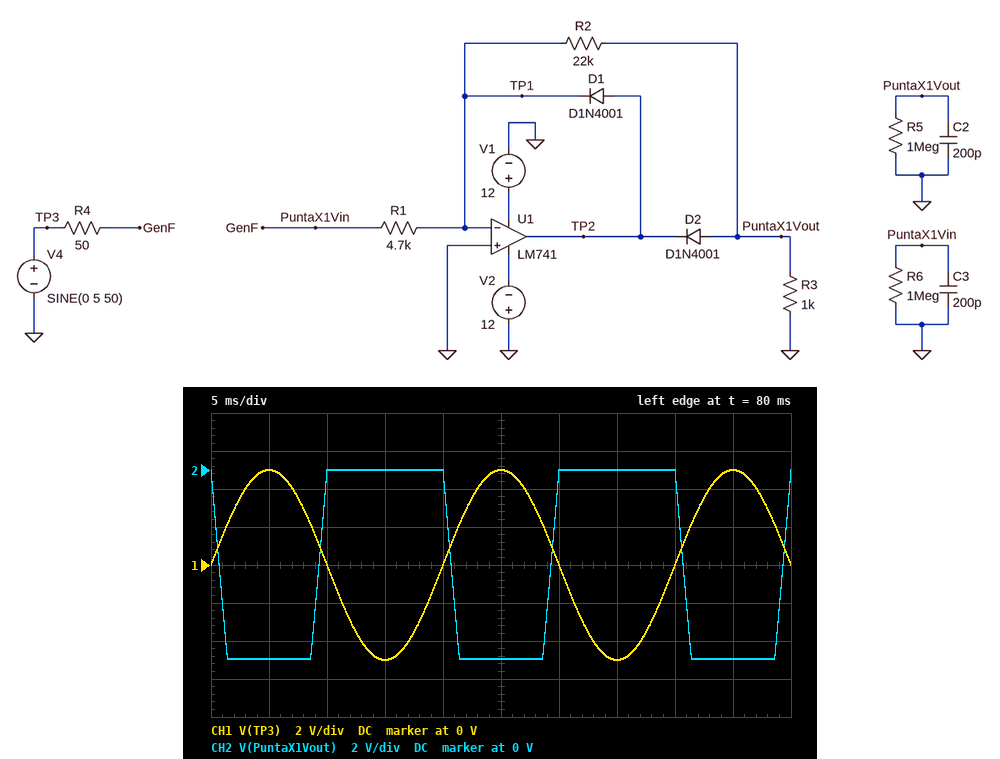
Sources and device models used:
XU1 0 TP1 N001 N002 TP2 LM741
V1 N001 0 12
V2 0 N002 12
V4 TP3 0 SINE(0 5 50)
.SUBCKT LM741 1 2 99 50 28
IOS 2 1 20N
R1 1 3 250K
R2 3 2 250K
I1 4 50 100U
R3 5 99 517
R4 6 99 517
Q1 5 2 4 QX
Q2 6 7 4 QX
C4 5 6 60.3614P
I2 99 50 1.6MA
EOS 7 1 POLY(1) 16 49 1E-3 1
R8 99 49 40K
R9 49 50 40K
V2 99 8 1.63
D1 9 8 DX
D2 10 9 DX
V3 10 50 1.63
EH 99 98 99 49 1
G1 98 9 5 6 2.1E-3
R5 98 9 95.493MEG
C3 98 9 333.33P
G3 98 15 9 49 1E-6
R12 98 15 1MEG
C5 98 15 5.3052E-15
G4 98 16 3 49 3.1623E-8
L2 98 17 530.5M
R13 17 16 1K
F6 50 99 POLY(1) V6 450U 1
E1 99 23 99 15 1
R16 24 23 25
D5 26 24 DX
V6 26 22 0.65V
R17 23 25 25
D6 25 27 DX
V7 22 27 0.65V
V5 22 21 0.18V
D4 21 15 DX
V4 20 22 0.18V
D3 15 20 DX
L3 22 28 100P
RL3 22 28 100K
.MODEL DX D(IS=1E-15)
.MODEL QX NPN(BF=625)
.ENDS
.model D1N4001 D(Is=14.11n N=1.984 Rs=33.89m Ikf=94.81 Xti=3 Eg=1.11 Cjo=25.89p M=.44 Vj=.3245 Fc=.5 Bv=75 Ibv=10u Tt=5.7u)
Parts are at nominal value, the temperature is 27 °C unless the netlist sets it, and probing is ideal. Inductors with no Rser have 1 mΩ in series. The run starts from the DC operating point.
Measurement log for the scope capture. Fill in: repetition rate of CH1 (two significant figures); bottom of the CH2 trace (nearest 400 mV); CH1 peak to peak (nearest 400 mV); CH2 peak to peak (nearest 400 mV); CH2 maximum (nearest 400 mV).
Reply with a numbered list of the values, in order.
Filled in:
1. 50 Hz
2. -10.0 V
3. 10.0 V
4. 10.0 V
5. 0 V
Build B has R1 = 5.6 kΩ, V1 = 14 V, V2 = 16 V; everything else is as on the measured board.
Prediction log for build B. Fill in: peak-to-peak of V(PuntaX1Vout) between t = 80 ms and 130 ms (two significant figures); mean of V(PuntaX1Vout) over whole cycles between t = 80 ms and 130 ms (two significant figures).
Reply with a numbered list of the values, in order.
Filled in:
1. 14 V
2. -5.3 V
